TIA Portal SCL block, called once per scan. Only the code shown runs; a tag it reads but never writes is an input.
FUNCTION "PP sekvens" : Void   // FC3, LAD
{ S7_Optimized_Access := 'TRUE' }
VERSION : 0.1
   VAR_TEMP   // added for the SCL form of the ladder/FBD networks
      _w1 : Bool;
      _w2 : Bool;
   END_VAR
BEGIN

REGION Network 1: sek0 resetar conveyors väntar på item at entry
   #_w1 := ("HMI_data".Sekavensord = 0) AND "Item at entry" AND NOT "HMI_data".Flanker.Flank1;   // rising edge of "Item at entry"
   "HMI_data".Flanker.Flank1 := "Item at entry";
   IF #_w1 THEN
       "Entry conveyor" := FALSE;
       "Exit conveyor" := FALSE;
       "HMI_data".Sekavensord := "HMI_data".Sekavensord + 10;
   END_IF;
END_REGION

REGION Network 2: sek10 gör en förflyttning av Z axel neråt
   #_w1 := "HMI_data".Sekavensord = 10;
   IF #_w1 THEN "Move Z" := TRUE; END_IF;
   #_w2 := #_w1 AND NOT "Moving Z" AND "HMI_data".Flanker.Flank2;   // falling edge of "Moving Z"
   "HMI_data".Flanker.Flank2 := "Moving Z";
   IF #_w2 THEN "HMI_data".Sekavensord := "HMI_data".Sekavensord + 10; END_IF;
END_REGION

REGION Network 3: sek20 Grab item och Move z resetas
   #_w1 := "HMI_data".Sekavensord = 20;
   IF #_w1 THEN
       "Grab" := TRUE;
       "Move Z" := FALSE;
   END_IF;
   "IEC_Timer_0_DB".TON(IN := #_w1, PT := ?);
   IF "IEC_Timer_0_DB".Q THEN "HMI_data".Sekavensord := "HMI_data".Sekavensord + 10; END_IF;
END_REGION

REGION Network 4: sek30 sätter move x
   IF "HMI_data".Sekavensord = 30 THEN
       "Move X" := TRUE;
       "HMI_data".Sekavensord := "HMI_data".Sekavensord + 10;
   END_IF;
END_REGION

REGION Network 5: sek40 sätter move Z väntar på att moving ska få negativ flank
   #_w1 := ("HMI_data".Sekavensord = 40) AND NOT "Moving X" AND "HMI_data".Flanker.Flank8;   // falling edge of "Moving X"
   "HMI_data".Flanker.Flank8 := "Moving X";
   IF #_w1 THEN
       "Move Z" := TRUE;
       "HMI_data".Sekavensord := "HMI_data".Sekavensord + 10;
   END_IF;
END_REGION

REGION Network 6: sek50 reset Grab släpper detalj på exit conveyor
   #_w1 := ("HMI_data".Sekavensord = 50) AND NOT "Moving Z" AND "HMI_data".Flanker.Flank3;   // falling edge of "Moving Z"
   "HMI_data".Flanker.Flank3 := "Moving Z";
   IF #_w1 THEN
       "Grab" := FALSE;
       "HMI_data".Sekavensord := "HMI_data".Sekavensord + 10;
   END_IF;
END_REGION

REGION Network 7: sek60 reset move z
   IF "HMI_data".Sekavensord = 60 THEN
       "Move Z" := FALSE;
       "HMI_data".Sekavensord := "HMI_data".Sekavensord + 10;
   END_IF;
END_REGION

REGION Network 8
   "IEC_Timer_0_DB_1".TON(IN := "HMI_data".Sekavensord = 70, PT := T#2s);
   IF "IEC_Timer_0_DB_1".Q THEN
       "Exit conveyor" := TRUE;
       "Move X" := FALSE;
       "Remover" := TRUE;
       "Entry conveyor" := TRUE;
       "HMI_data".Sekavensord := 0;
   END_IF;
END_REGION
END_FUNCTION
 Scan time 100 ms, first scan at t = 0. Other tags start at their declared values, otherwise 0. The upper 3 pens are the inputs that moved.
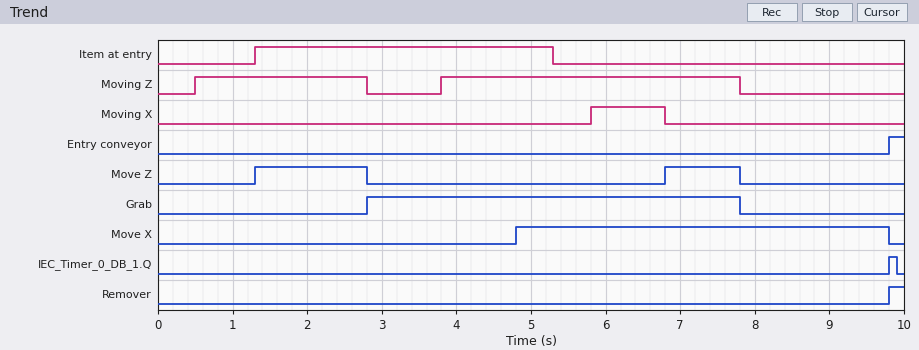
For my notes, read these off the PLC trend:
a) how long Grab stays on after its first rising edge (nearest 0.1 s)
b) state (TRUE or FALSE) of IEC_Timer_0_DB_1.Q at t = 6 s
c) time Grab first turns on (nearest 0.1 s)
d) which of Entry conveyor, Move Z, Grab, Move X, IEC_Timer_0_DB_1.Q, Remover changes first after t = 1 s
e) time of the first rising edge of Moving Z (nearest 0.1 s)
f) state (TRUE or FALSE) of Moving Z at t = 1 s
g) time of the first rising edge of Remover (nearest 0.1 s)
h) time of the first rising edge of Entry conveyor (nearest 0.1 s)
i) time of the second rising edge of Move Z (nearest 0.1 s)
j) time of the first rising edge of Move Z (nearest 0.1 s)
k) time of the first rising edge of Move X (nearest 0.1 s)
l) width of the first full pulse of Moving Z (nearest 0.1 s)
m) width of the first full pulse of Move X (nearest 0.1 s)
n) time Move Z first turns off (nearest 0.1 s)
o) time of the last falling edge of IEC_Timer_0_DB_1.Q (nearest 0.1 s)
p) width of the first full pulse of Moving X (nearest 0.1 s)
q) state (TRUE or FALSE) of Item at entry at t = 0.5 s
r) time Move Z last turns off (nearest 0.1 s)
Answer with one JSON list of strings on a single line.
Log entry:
["5.0 s", "FALSE", "2.8 s", "Move Z", "0.5 s", "TRUE", "9.8 s", "9.8 s", "6.8 s", "1.3 s", "4.8 s", "2.3 s", "5.0 s", "2.8 s", "9.9 s", "1.0 s", "FALSE", "7.8 s"]
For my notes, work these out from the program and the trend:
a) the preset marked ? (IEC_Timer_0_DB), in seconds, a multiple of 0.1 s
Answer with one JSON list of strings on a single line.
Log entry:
["2.0 s"]
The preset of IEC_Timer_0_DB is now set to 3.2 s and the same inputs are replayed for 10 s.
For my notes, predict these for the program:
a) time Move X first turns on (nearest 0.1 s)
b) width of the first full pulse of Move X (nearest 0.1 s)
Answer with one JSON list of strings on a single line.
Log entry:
["6.0 s", "3.8 s"]
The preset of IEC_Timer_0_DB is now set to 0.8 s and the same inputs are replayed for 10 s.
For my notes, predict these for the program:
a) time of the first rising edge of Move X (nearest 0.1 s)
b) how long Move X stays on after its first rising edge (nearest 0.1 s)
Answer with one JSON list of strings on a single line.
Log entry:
["3.6 s", "6.2 s"]
